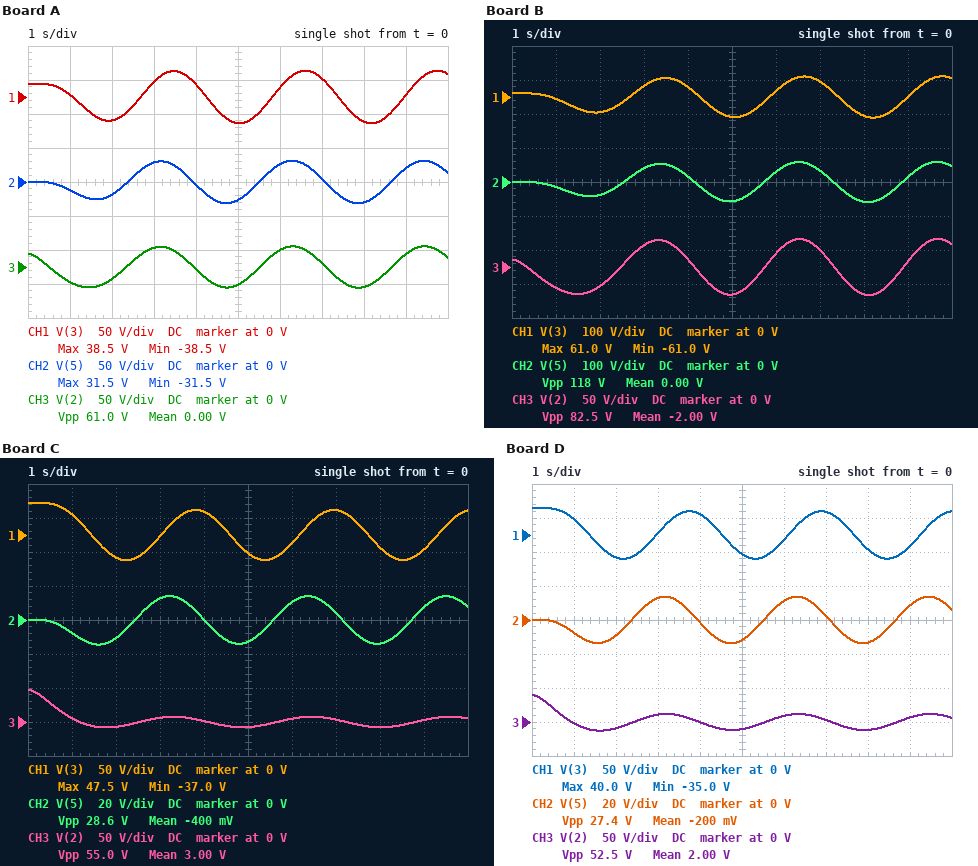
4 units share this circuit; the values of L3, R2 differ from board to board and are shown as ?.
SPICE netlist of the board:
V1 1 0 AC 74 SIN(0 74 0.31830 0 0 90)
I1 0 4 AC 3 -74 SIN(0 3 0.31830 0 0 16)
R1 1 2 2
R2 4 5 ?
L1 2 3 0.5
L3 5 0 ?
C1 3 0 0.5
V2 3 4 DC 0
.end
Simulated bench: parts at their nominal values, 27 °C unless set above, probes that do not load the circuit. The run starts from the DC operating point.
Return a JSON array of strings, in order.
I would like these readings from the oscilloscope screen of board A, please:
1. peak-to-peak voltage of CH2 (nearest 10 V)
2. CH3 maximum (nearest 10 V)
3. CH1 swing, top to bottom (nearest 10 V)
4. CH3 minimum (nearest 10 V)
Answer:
["60 V", "30 V", "80 V", "-30 V"]
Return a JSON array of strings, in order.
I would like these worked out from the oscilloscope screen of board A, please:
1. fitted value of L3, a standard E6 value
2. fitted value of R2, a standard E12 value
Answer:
["470 mH", "0.68 Ω"]
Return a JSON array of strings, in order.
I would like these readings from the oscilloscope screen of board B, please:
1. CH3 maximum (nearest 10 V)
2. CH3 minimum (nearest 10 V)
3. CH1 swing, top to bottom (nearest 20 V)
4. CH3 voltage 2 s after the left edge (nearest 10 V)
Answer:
["40 V", "-40 V", "120 V", "-30 V"]
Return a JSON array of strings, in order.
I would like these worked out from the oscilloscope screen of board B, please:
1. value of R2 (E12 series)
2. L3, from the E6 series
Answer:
["0.33 Ω", "680 mH"]
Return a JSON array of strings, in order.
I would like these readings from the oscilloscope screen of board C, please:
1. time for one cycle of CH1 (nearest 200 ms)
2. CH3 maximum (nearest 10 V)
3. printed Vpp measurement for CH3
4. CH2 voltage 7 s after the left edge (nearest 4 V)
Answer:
["3.2 s", "50 V", "55.0 V", "4 V"]
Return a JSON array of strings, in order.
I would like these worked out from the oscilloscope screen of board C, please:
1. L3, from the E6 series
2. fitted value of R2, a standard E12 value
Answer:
["680 mH", "3.3 Ω"]
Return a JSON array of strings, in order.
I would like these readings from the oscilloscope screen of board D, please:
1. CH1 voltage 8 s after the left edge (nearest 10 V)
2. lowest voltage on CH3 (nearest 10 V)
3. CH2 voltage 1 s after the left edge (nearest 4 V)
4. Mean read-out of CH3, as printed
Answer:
["-20 V", "-10 V", "-8 V", "2.00 V"]
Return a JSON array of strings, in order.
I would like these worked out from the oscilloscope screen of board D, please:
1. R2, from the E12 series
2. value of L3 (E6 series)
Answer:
["2.2 Ω", "470 mH"]
